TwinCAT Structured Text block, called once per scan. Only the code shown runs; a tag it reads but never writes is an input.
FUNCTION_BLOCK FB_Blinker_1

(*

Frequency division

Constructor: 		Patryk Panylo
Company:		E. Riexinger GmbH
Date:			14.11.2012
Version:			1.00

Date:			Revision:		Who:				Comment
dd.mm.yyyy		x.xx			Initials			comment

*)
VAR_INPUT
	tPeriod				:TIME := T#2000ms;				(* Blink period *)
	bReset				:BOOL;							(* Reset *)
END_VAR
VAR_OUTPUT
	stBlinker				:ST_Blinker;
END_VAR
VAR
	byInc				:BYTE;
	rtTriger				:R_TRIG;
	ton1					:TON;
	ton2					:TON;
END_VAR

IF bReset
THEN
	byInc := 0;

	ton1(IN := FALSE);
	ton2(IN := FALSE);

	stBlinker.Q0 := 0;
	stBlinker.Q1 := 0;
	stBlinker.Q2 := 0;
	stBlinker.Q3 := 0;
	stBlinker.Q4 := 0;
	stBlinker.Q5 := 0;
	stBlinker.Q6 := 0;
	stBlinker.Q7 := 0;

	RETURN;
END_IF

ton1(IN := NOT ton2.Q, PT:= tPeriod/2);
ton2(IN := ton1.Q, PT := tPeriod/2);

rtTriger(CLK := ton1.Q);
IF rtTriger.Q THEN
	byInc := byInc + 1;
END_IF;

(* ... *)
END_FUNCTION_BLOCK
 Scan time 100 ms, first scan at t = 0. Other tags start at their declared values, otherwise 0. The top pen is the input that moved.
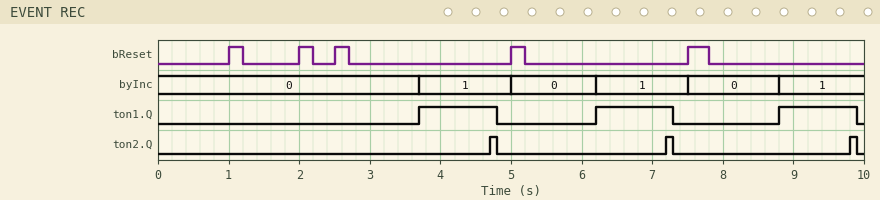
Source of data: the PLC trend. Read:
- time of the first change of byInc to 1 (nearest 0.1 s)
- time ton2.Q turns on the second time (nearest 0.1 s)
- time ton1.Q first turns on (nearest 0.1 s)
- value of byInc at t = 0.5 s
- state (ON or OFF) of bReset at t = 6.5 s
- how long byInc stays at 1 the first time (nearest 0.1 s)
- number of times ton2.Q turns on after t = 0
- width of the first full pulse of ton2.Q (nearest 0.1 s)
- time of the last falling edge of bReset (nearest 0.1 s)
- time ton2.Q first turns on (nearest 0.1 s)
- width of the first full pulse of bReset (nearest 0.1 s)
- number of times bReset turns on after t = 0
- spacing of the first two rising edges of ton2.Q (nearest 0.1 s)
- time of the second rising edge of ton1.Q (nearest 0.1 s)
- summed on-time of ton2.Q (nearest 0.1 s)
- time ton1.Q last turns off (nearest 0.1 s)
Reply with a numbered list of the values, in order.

1. 3.7 s
2. 7.2 s
3. 3.7 s
4. 0
5. OFF
6. 1.3 s
7. 3
8. 0.1 s
9. 7.8 s
10. 4.7 s
11. 0.2 s
12. 5
13. 2.5 s
14. 6.2 s
15. 0.3 s
16. 9.9 s
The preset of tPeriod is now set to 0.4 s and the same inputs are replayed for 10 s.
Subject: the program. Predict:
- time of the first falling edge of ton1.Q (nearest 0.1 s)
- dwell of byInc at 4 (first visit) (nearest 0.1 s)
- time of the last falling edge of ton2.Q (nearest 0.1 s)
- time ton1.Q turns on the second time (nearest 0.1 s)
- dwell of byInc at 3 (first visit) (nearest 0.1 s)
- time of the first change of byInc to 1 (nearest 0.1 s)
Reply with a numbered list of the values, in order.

1. 0.5 s
2. 0.3 s
3. 9.5 s
4. 0.8 s
5. 0.6 s
6. 0.2 s
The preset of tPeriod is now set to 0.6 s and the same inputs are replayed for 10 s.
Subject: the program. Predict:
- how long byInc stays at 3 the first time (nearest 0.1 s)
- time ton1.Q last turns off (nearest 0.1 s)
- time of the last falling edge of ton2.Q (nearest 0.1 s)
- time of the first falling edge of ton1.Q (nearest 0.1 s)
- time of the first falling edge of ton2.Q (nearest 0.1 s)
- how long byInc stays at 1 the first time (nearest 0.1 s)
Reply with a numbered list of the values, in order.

1. 0.4 s
2. 9.3 s
3. 9.3 s
4. 0.7 s
5. 0.7 s
6. 0.7 s
